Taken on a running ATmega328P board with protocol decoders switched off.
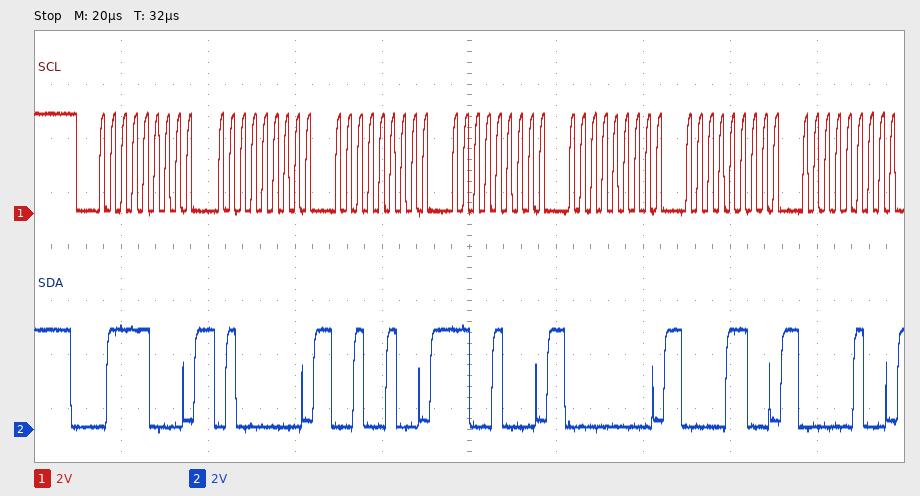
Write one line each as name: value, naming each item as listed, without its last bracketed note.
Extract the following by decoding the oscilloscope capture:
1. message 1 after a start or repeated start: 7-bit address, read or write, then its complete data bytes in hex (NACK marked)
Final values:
message 1 after a start or repeated start: 7-bit address, read or write, then its complete data bytes in hex: 0x3C write: 40 24 C8 00 0C 04
